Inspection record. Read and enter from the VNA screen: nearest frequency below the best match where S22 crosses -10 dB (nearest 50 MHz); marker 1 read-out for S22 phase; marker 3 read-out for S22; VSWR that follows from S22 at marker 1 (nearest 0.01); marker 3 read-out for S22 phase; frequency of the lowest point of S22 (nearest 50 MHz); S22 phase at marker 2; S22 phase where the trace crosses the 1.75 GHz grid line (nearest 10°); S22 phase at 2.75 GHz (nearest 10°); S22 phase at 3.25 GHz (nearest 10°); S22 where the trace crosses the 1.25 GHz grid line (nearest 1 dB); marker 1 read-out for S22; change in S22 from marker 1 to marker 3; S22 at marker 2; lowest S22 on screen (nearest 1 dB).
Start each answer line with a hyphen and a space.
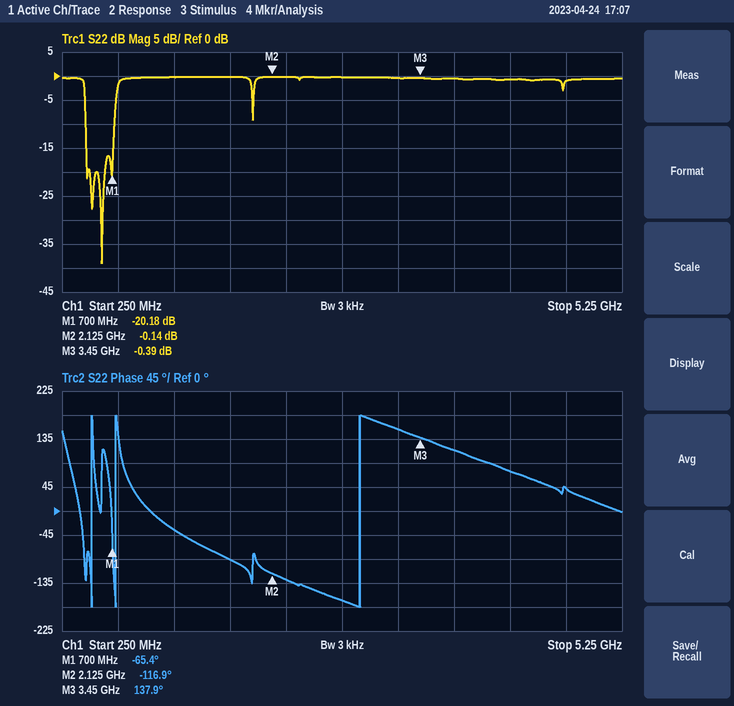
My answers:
- 450 MHz
- -65.4°
- -0.39 dB
- 1.22
- 137.9°
- 600 MHz
- -116.9°
- -90°
- -170°
- 150°
- 0 dB
- -20.18 dB
- 19.79 dB
- -0.14 dB
- -39 dB
